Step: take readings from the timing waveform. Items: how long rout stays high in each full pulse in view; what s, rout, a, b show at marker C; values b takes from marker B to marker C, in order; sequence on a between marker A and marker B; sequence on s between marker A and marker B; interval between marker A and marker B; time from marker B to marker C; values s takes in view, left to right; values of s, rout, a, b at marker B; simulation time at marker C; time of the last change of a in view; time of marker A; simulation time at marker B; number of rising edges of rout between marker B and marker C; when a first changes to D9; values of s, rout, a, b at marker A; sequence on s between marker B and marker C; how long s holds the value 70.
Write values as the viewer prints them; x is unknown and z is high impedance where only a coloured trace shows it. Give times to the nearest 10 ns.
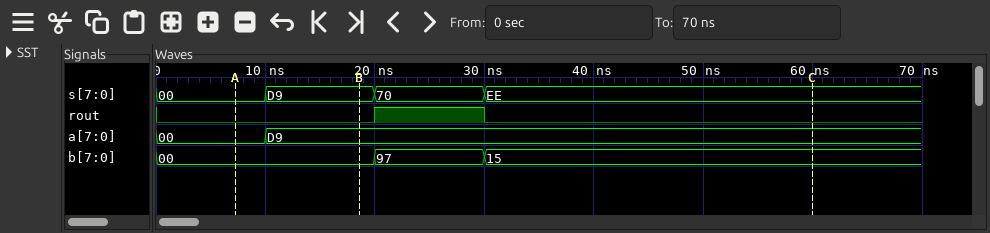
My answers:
10 ns
s=EE, rout=0, a=D9, b=15
00, 97, 15
00, D9
00, D9
10 ns
40 ns
00, D9, 70, EE
s=D9, rout=0, a=D9, b=00
60 ns
10 ns
10 ns
20 ns
1
10 ns
s=00, rout=0, a=00, b=00
D9, 70, EE
10 ns
